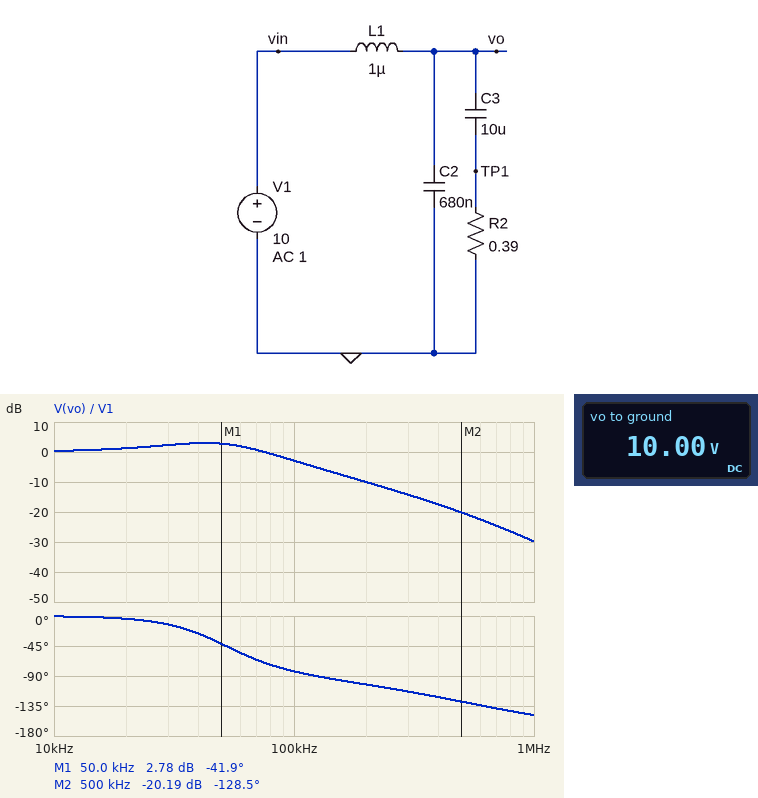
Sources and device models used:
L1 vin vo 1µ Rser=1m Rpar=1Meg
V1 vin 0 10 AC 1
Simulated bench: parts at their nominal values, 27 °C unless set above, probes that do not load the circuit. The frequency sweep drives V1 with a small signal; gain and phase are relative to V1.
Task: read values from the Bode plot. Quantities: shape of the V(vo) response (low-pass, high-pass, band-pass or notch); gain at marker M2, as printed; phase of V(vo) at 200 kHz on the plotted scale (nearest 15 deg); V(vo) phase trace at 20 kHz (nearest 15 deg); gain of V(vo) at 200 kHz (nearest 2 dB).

low-pass
-20.19 dB
-105 deg
0 deg
-10 dB
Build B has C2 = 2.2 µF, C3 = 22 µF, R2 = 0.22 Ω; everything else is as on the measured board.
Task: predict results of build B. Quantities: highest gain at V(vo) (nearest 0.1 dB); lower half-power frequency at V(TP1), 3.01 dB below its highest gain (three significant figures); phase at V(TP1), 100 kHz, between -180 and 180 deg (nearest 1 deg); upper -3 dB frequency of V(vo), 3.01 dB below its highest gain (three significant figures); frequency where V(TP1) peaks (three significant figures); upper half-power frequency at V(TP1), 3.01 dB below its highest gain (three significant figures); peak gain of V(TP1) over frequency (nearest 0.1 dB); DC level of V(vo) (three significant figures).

4.0 dB
21.5 kHz
-87 deg
46.0 kHz
33.8 kHz
52.8 kHz
0.8 dB
10.0 V
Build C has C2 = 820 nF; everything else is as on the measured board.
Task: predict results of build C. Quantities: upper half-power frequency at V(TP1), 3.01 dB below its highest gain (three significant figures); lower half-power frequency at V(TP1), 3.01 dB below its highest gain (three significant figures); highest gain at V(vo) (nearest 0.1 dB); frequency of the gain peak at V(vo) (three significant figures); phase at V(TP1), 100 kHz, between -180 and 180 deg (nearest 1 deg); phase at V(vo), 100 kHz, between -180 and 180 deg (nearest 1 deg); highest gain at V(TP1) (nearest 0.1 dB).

87.8 kHz
29.5 kHz
3.1 dB
43.3 kHz
-63 deg
-85 deg
0.7 dB
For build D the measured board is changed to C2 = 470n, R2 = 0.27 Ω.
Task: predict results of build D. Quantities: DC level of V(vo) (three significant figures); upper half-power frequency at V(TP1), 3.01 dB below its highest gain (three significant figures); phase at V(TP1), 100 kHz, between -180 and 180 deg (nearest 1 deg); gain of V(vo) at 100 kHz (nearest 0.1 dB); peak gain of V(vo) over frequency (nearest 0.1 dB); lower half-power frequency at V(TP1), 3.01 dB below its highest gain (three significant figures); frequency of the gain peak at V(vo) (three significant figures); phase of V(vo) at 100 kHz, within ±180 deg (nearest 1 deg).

10.0 V
74.1 kHz
-66 deg
-4.8 dB
4.4 dB
33.6 kHz
44.7 kHz
-97 deg
